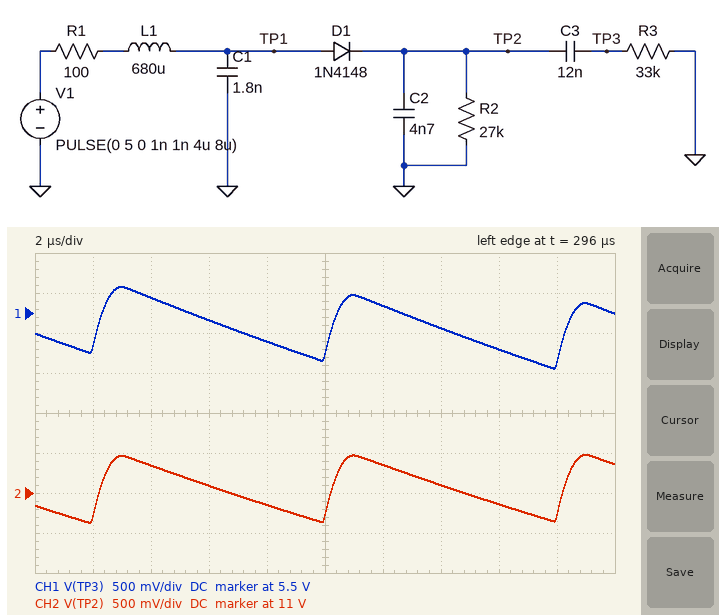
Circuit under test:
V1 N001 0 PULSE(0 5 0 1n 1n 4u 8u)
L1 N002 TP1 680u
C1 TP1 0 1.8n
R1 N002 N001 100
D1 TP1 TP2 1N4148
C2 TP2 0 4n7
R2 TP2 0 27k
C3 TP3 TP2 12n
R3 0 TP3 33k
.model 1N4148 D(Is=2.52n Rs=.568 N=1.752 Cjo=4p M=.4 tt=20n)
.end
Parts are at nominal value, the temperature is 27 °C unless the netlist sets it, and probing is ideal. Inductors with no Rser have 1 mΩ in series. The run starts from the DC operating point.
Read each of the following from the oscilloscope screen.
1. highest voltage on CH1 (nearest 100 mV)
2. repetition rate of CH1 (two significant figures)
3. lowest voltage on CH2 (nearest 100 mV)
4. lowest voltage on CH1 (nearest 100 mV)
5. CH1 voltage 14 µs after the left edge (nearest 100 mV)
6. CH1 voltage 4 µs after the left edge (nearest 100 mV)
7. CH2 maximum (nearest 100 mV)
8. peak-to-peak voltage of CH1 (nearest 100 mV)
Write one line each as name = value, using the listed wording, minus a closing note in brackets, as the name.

highest voltage on CH1 = 5.8 V
repetition rate of CH1 = 120 kHz
lowest voltage on CH2 = 10.6 V
lowest voltage on CH1 = 4.8 V
CH1 voltage 14 µs after the left edge = 5.3 V
CH1 voltage 4 µs after the left edge = 5.7 V
CH2 maximum = 11.5 V
peak-to-peak voltage of CH1 = 1.0 V
